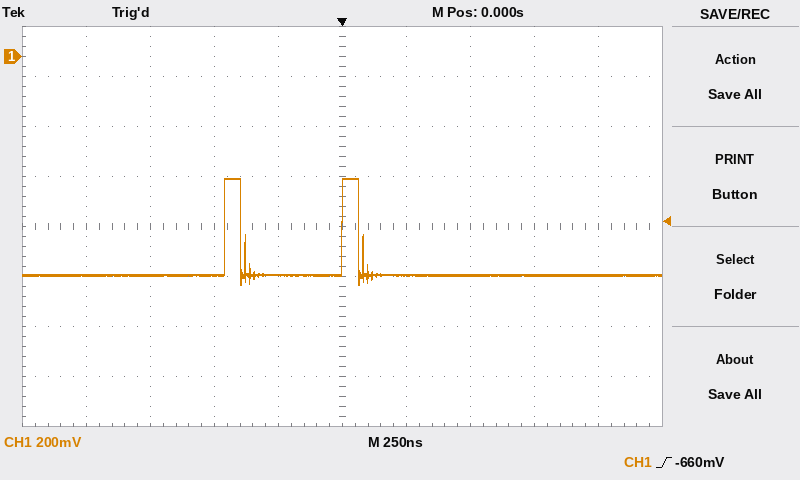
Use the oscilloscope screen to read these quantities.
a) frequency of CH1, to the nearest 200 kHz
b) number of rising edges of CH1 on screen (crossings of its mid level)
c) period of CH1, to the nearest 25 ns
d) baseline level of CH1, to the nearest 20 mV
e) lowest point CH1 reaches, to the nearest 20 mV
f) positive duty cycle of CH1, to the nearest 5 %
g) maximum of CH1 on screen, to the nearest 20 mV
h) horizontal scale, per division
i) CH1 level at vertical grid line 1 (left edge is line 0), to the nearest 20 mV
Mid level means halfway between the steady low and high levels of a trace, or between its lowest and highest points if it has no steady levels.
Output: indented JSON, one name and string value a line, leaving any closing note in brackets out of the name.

{
  "frequency of CH1, to the nearest 200 kHz": "2.2 MHz",
  "number of rising edges of CH1 on screen": "2",
  "period of CH1, to the nearest 25 ns": "450 ns",
  "baseline level of CH1, to the nearest 20 mV": "-880 mV",
  "lowest point CH1 reaches, to the nearest 20 mV": "-920 mV",
  "positive duty cycle of CH1, to the nearest 5 %": "15 %",
  "maximum of CH1 on screen, to the nearest 20 mV": "-480 mV",
  "horizontal scale, per division": "250 ns",
  "CH1 level at vertical grid line 1 (left edge is line 0), to the nearest 20 mV": "-880 mV"
}
